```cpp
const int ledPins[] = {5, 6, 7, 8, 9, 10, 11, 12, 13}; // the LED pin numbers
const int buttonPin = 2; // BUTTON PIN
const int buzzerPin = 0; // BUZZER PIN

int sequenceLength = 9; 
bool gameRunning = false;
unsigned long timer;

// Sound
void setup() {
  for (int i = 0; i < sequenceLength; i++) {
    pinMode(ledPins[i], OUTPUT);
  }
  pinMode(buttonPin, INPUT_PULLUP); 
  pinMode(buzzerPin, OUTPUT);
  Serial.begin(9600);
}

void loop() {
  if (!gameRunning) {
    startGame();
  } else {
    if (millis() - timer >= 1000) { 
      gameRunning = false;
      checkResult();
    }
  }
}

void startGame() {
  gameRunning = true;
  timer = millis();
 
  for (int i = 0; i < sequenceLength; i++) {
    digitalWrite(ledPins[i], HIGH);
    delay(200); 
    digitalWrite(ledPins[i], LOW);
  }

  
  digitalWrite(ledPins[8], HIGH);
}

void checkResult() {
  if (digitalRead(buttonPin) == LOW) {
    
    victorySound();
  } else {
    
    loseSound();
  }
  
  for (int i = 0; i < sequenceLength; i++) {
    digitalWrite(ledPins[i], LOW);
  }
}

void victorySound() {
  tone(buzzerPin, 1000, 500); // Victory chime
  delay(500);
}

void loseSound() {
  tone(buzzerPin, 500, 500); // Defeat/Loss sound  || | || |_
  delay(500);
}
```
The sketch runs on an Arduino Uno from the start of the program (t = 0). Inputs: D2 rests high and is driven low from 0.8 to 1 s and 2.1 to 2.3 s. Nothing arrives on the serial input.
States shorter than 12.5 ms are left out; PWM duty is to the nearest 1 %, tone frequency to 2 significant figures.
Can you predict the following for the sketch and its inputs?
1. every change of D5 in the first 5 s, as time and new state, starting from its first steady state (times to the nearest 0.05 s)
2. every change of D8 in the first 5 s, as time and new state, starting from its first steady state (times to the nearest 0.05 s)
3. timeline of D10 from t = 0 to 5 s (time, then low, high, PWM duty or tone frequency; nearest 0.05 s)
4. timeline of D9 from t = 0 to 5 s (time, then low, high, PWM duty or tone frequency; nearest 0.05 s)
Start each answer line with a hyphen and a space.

- 0 s high; 0.2 s low; 2.3 s high; 2.5 s low; 4.6 s high; 4.8 s low
- 0 s low; 0.6 s high; 0.8 s low; 2.9 s high; 3.1 s low
- 0 s low; 1 s high; 1.2 s low; 3.3 s high; 3.5 s low
- 0 s low; 0.8 s high; 1 s low; 3.1 s high; 3.3 s low
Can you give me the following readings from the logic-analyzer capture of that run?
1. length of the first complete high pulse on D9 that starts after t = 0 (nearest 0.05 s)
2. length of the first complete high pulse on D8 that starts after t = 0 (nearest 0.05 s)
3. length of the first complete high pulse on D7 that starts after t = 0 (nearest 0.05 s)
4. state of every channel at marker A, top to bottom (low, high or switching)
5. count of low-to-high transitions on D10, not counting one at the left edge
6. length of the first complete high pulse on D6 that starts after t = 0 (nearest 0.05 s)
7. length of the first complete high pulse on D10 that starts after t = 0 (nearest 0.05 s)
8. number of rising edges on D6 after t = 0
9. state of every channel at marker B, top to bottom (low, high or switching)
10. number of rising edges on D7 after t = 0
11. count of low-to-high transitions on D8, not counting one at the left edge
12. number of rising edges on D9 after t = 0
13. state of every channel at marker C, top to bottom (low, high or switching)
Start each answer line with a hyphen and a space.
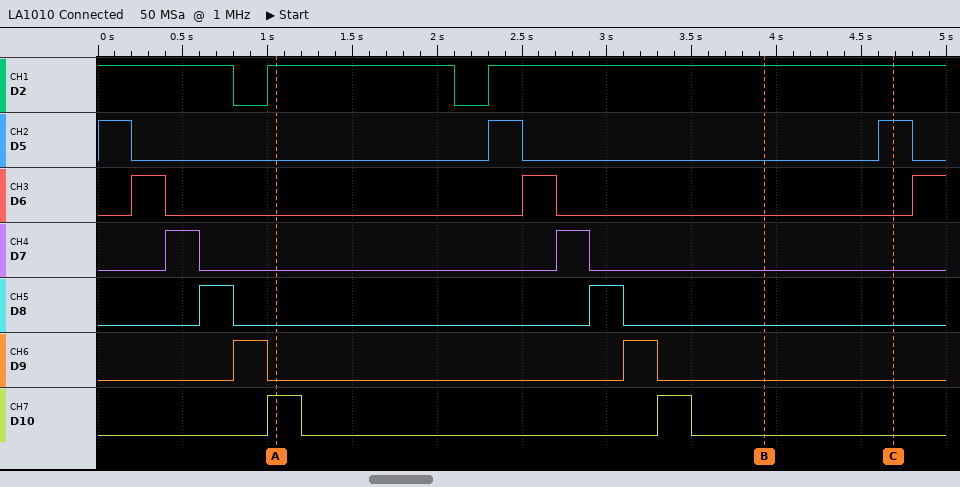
- 0.20 s
- 0.20 s
- 0.20 s
- D2 high, D5 low, D6 low, D7 low, D8 low, D9 low, D10 high
- 2
- 0.20 s
- 0.20 s
- 3
- D2 high, D5 low, D6 low, D7 low, D8 low, D9 low, D10 low
- 2
- 2
- 2
- D2 high, D5 high, D6 low, D7 low, D8 low, D9 low, D10 low
